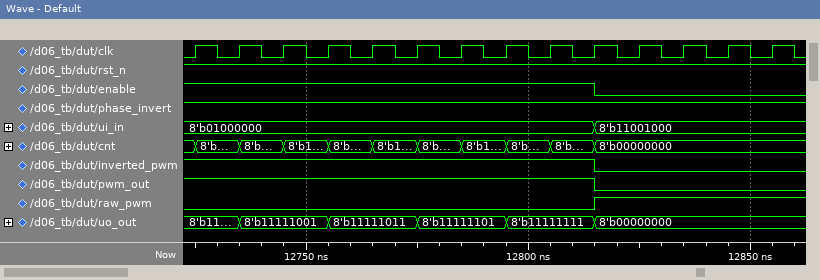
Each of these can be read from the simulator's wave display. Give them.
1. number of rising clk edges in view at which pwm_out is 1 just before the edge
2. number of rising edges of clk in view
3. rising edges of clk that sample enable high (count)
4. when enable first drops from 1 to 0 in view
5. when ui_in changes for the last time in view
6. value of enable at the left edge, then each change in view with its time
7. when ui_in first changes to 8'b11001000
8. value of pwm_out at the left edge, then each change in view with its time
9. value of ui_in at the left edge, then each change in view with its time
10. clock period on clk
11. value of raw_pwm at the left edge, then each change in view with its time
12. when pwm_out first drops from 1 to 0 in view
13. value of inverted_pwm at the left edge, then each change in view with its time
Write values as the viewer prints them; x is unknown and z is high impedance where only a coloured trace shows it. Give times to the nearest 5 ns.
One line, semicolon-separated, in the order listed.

10; 14; 10; 12815 ns; 12815 ns; 1, 0 at 12815 ns; 12815 ns; 1, 0 at 12815 ns; 8'b01000000, 8'b11001000 at 12815 ns; 10 ns; 0, 1 at 12815 ns; 12815 ns; 1, 0 at 12815 ns
